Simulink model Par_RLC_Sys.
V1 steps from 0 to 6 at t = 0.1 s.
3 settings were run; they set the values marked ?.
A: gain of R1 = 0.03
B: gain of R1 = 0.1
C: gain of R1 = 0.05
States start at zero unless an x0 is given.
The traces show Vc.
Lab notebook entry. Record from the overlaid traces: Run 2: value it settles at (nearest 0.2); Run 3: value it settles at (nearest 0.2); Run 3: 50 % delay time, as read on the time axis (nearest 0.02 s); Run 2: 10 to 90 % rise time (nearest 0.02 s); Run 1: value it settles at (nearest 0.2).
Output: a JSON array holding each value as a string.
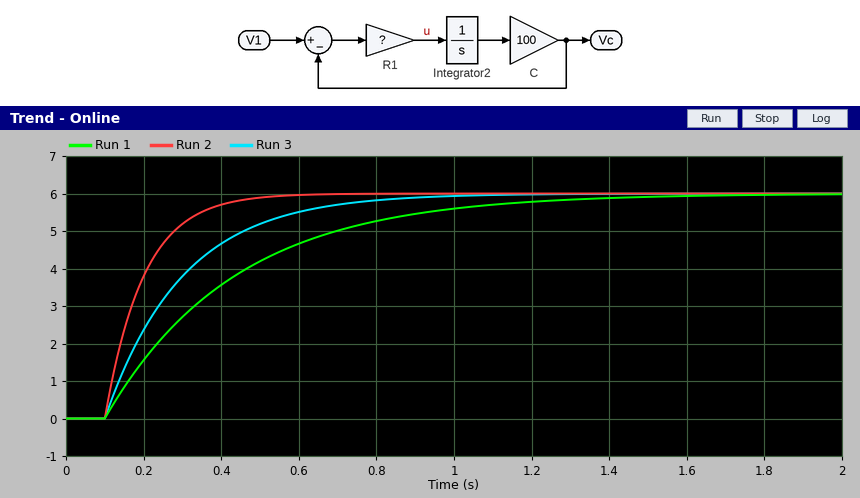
["6.0", "6.0", "0.24 s", "0.22 s", "6.0"]
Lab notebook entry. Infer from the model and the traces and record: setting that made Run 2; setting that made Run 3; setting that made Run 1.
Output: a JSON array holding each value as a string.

["B", "C", "A"]
